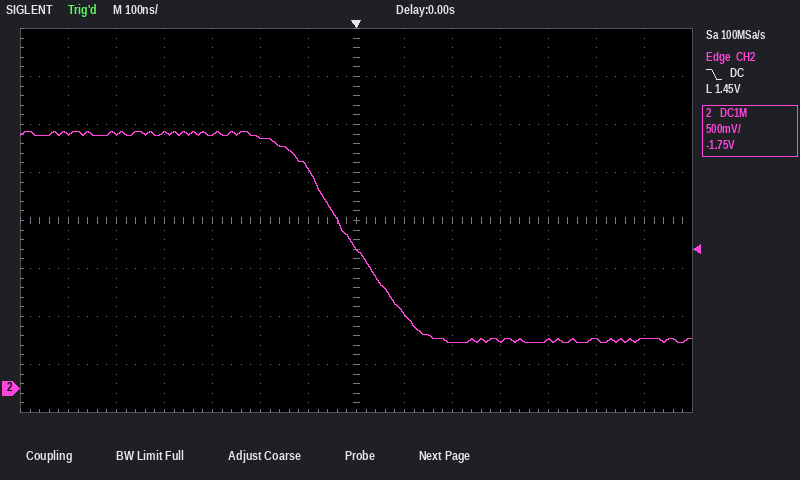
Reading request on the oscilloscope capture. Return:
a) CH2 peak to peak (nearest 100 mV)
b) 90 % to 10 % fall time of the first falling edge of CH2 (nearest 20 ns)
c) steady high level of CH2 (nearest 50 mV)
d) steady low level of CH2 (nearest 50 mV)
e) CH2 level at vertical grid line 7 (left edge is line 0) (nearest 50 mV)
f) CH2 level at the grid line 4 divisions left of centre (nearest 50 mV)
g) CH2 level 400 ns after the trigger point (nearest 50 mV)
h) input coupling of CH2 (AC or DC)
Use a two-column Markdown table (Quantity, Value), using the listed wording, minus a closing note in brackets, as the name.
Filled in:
| Quantity | Value |
|---|---|
| CH2 peak to peak | 2.20 V |
| 90 % to 10 % fall time of the first falling edge of CH2 | 240 ns |
| steady high level of CH2 | 2.65 V |
| steady low level of CH2 | 500 mV |
| CH2 level at vertical grid line 7 (left edge is line 0) | 1.45 V |
| CH2 level at the grid line 4 divisions left of centre | 2.65 V |
| CH2 level 400 ns after the trigger point | 500 mV |
| input coupling of CH2 | DC |
